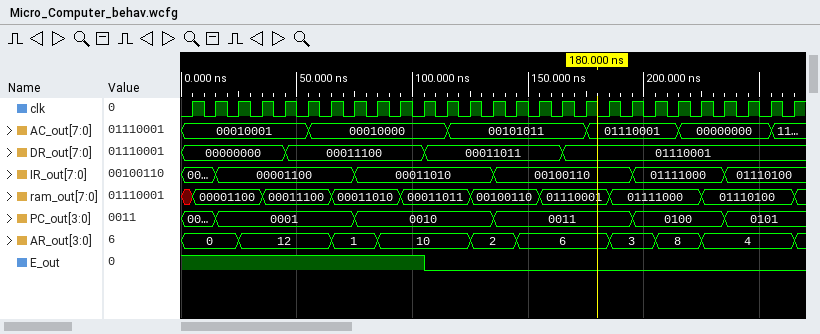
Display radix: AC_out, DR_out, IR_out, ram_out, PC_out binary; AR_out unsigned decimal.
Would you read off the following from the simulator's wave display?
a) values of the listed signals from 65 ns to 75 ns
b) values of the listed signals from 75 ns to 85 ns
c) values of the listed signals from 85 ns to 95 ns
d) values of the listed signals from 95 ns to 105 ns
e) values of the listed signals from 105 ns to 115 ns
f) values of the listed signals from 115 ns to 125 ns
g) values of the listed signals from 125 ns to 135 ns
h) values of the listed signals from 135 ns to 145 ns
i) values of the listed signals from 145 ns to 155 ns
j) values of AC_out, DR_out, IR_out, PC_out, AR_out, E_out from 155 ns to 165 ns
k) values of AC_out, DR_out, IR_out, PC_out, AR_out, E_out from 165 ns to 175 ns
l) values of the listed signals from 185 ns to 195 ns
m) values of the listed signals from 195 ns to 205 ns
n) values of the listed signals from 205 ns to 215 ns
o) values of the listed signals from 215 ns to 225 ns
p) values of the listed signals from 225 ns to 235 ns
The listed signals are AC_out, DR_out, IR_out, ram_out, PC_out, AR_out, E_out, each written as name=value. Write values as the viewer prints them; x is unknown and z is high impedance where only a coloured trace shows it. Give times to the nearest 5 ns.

AC_out=00010000, DR_out=00011100, IR_out=00001100, ram_out=00011010, PC_out=0001, AR_out=1, E_out=1
AC_out=00010000, DR_out=00011100, IR_out=00011010, ram_out=00011010, PC_out=0010, AR_out=1, E_out=1
AC_out=00010000, DR_out=00011100, IR_out=00011010, ram_out=00011010, PC_out=0010, AR_out=10, E_out=1
AC_out=00010000, DR_out=00011100, IR_out=00011010, ram_out=00011011, PC_out=0010, AR_out=10, E_out=1
AC_out=00010000, DR_out=00011011, IR_out=00011010, ram_out=00011011, PC_out=0010, AR_out=10, E_out=0
AC_out=00101011, DR_out=00011011, IR_out=00011010, ram_out=00011011, PC_out=0010, AR_out=10, E_out=0
AC_out=00101011, DR_out=00011011, IR_out=00011010, ram_out=00100110, PC_out=0010, AR_out=2, E_out=0
AC_out=00101011, DR_out=00011011, IR_out=00100110, ram_out=00100110, PC_out=0011, AR_out=2, E_out=0
AC_out=00101011, DR_out=00011011, IR_out=00100110, ram_out=00100110, PC_out=0011, AR_out=6, E_out=0
AC_out=00101011, DR_out=00011011, IR_out=00100110, PC_out=0011, AR_out=6, E_out=0
AC_out=00101011, DR_out=01110001, IR_out=00100110, PC_out=0011, AR_out=6, E_out=0
AC_out=01110001, DR_out=01110001, IR_out=00100110, ram_out=01111000, PC_out=0011, AR_out=3, E_out=0
AC_out=01110001, DR_out=01110001, IR_out=01111000, ram_out=01111000, PC_out=0100, AR_out=3, E_out=0
AC_out=01110001, DR_out=01110001, IR_out=01111000, ram_out=01111000, PC_out=0100, AR_out=8, E_out=0
AC_out=00000000, DR_out=01110001, IR_out=01111000, ram_out=01111000, PC_out=0100, AR_out=8, E_out=0
AC_out=00000000, DR_out=01110001, IR_out=01111000, ram_out=01110100, PC_out=0100, AR_out=4, E_out=0
